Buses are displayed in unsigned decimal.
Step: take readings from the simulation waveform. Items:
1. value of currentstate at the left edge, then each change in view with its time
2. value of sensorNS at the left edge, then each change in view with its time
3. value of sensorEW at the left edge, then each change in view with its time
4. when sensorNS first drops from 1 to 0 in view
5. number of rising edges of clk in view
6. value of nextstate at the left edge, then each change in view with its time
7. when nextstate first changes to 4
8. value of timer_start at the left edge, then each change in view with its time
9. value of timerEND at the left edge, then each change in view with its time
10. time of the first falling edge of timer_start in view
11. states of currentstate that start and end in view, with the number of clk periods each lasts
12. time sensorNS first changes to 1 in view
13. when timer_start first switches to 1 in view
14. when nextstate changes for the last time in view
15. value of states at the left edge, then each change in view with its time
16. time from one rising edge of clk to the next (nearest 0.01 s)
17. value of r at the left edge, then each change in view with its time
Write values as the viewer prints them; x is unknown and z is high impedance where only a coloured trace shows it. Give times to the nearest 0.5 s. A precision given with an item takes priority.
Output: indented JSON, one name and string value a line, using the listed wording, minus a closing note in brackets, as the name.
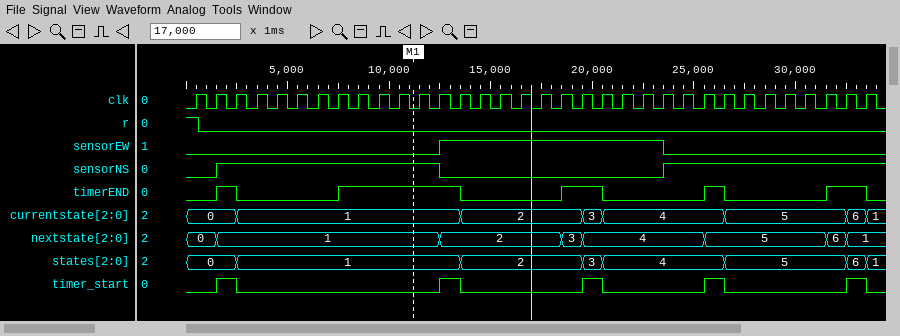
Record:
{
  "value of currentstate at the left edge, then each change in view with its time": "0, 1 at 2.5 s, 2 at 13.5 s, 3 at 19.5 s, 4 at 20.5 s, 5 at 26.5 s, 6 at 32.5 s, 1 at 33.5 s",
  "value of sensorNS at the left edge, then each change in view with its time": "0, 1 at 1.5 s, 0 at 12.5 s, 1 at 23.5 s",
  "value of sensorEW at the left edge, then each change in view with its time": "0, 1 at 12.5 s, 0 at 23.5 s",
  "when sensorNS first drops from 1 to 0 in view": "12.5 s",
  "number of rising edges of clk in view": "34",
  "value of nextstate at the left edge, then each change in view with its time": "0, 1 at 1.5 s, 2 at 12.5 s, 3 at 18.5 s, 4 at 19.5 s, 5 at 25.5 s, 6 at 31.5 s, 1 at 32.5 s",
  "when nextstate first changes to 4": "19.5 s",
  "value of timer_start at the left edge, then each change in view with its time": "0, 1 at 1.5 s, 0 at 2.5 s, 1 at 12.5 s, 0 at 13.5 s, 1 at 19.5 s, 0 at 20.5 s, 1 at 25.5 s, 0 at 26.5 s, 1 at 32.5 s, 0 at 33.5 s",
  "value of timerEND at the left edge, then each change in view with its time": "0, 1 at 1.5 s, 0 at 2.5 s, 1 at 7.5 s, 0 at 13.5 s, 1 at 18.5 s, 0 at 20.5 s, 1 at 25.5 s, 0 at 26.5 s, 1 at 31.5 s, 0 at 33.5 s",
  "time of the first falling edge of timer_start in view": "2.5 s",
  "states of currentstate that start and end in view, with the number of clk periods each lasts": "1: 11, 2: 6, 3: 1, 4: 6, 5: 6, 6: 1",
  "time sensorNS first changes to 1 in view": "1.5 s",
  "when timer_start first switches to 1 in view": "1.5 s",
  "when nextstate changes for the last time in view": "32.5 s",
  "value of states at the left edge, then each change in view with its time": "0, 1 at 2.5 s, 2 at 13.5 s, 3 at 19.5 s, 4 at 20.5 s, 5 at 26.5 s, 6 at 32.5 s, 1 at 33.5 s",
  "time from one rising edge of clk to the next": "1 s",
  "value of r at the left edge, then each change in view with its time": "1, 0 at 0.5 s"
}
